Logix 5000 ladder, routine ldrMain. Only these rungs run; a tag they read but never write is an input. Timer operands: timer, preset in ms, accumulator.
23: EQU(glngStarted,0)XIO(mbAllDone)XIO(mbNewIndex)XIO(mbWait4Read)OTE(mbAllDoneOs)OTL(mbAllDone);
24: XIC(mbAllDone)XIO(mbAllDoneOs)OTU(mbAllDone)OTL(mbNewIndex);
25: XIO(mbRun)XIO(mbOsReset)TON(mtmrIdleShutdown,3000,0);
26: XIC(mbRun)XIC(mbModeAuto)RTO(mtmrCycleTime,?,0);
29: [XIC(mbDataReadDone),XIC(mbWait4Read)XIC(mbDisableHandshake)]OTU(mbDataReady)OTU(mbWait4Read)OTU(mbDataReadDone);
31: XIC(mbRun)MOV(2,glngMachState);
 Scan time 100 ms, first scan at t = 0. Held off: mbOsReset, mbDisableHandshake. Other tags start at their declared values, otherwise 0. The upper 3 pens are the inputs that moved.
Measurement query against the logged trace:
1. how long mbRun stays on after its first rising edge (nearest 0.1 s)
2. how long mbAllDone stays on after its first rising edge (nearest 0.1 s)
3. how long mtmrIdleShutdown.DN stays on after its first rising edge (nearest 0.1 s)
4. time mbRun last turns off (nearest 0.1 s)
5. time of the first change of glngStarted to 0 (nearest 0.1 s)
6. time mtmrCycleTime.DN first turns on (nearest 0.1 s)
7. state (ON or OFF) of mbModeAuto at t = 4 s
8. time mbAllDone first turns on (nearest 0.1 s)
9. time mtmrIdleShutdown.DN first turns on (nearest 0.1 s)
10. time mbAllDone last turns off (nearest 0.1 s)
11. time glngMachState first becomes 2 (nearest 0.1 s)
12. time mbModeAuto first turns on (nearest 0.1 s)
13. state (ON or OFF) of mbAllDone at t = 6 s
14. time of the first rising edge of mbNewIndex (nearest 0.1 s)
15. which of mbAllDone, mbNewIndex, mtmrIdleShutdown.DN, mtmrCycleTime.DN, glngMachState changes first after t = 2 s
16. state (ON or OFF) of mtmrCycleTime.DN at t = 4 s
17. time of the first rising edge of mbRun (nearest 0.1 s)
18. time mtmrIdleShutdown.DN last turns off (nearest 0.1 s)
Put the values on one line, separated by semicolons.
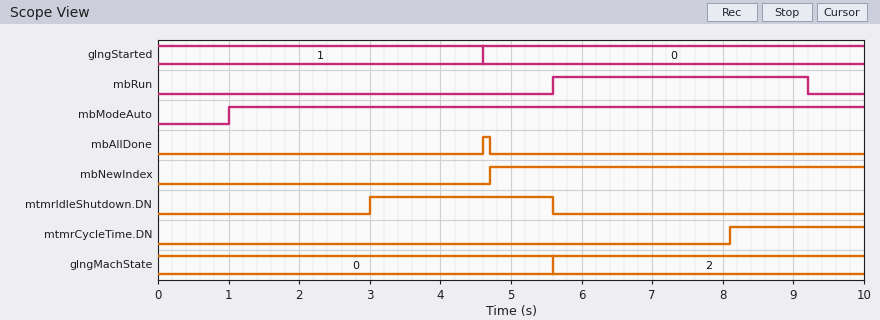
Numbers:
3.6 s; 0.1 s; 2.6 s; 9.2 s; 4.6 s; 8.1 s; ON; 4.6 s; 3.0 s; 4.7 s; 5.6 s; 1.0 s; OFF; 4.7 s; mtmrIdleShutdown.DN; OFF; 5.6 s; 5.6 s
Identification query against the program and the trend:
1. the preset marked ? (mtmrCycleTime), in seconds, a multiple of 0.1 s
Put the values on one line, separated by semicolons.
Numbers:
2.5 s
